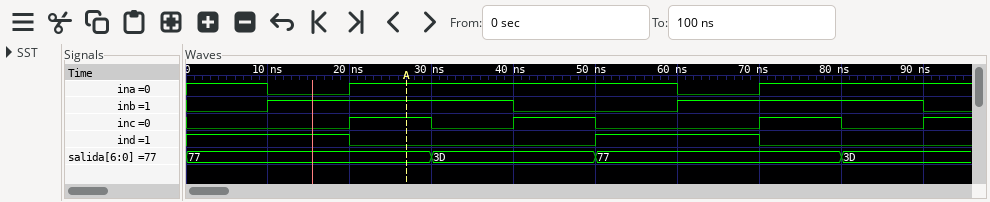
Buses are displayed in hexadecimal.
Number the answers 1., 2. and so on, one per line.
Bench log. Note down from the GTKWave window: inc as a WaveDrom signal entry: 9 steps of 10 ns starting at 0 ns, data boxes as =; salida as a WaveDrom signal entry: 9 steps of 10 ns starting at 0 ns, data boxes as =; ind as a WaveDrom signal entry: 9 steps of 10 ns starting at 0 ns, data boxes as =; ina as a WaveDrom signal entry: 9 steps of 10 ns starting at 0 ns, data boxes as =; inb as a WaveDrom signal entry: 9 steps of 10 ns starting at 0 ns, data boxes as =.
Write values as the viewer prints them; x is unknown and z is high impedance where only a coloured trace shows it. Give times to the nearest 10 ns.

1. {name: 'inc', wave: '0.1010.10'}
2. {name: 'salida', wave: '=..=.=..=', data: '77 3D 77 3D'}
3. {name: 'ind', wave: '1.0..1.0.'}
4. {name: 'ina', wave: '101...01.'}
5. {name: 'inb', wave: '01..0.1..'}
